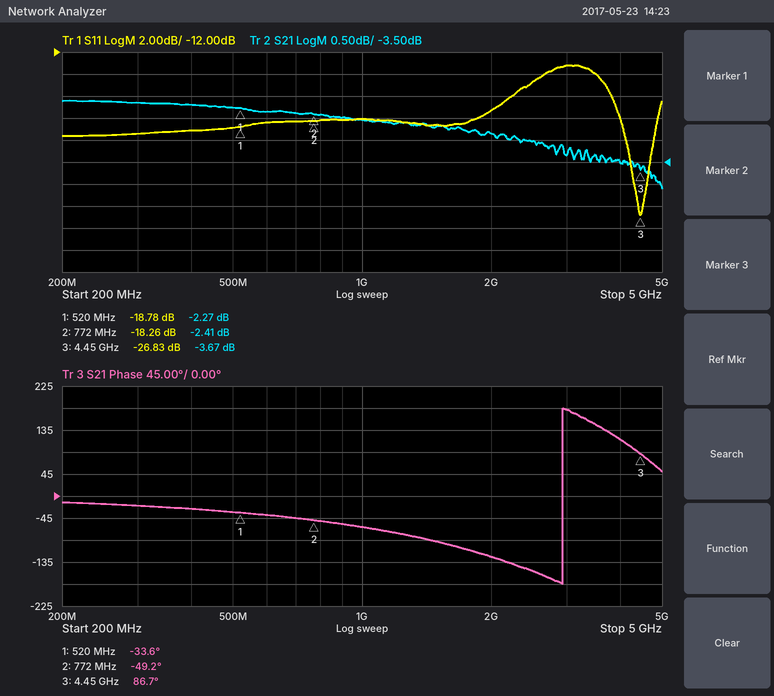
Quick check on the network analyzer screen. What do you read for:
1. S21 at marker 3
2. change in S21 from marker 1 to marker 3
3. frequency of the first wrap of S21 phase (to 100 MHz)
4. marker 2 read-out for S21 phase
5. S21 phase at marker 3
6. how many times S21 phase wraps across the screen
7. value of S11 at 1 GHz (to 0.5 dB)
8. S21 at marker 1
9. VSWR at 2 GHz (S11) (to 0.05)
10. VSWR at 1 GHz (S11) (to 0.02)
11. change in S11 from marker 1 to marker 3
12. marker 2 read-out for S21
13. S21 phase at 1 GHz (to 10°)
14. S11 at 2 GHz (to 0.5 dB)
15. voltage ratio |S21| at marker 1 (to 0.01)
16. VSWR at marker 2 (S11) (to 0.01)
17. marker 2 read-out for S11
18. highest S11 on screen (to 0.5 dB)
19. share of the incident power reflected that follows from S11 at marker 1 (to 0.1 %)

-3.67 dB
-1.40 dB
2.9 GHz
-49.2°
86.7°
1
-18.0 dB
-2.27 dB
1.30
1.28
-8.05 dB
-2.41 dB
-60°
-17.5 dB
0.77
1.28
-18.26 dB
-13.0 dB
1.3 %
